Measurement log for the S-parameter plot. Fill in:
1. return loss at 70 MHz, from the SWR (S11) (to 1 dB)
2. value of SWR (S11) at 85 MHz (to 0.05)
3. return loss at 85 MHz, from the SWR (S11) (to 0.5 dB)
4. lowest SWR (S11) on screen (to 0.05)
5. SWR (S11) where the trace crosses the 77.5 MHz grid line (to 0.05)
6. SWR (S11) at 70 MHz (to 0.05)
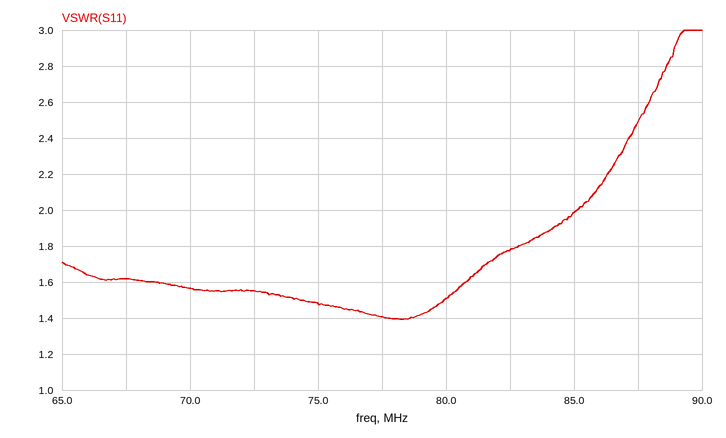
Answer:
13 dB
2.00
9.5 dB
1.40
1.40
1.55
